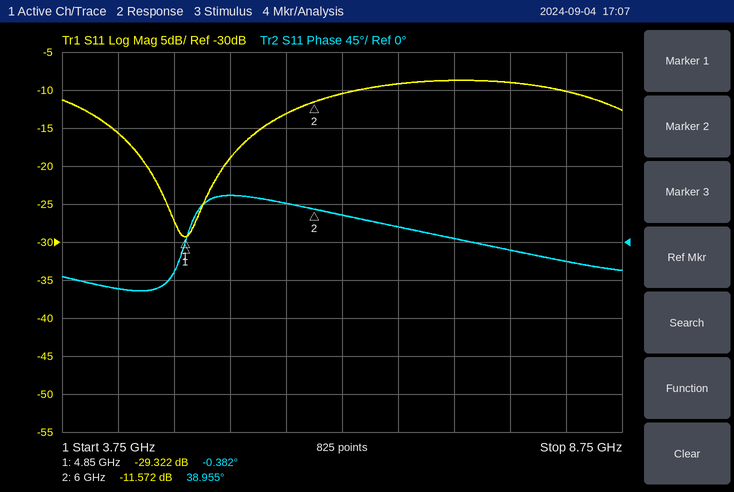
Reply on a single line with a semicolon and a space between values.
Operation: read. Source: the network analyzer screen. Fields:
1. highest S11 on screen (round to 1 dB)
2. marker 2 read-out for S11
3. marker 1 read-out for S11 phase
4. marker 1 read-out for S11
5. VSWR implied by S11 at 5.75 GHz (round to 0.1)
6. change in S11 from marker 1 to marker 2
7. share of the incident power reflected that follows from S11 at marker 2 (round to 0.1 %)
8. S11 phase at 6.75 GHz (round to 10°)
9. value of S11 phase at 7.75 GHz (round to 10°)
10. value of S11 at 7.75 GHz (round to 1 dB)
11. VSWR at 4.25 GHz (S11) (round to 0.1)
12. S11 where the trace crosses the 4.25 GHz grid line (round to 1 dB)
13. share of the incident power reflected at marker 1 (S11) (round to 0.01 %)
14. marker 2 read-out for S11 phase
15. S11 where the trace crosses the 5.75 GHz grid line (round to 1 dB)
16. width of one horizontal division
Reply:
-9 dB; -11.572 dB; -0.382°; -29.322 dB; 1.6; 17.750 dB; 7.0 %; 20°; -10°; -9 dB; 1.4; -16 dB; 0.12 %; 38.955°; -13 dB; 500 MHz
